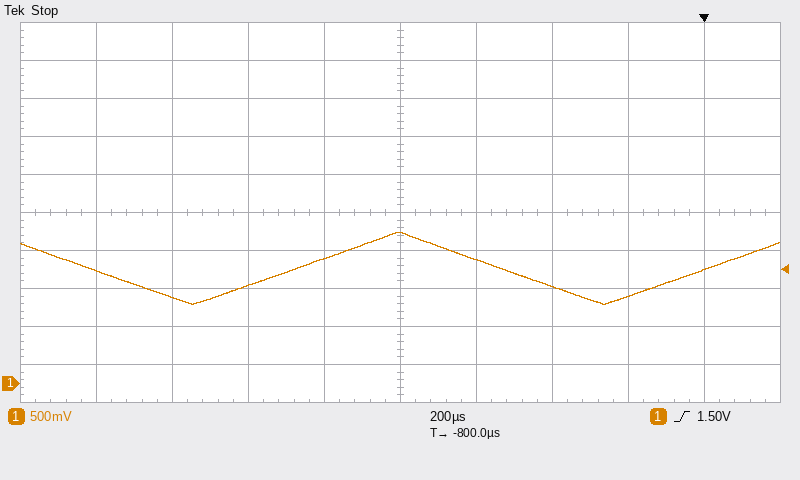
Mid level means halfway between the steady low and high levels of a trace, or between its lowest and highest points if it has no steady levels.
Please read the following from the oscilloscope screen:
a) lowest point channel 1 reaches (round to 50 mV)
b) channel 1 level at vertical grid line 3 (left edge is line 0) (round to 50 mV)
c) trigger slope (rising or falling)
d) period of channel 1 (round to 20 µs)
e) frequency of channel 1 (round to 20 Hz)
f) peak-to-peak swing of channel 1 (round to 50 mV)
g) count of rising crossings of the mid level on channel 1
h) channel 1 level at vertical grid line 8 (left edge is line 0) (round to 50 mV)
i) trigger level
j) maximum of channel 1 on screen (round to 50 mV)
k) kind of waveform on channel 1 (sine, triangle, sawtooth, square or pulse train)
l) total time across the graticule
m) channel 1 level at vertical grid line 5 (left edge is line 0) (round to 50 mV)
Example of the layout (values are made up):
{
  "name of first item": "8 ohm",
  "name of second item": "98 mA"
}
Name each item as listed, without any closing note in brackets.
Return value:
{
  "lowest point channel 1 reaches": "1.05 V",
  "channel 1 level at vertical grid line 3 (left edge is line 0)": "1.30 V",
  "trigger slope": "rising",
  "period of channel 1": "1.08 ms",
  "frequency of channel 1": "920 Hz",
  "peak-to-peak swing of channel 1": "950 mV",
  "count of rising crossings of the mid level on channel 1": "2",
  "channel 1 level at vertical grid line 8 (left edge is line 0)": "1.15 V",
  "trigger level": "1.50 V",
  "maximum of channel 1 on screen": "2.00 V",
  "kind of waveform on channel 1": "triangle",
  "total time across the graticule": "2 ms",
  "channel 1 level at vertical grid line 5 (left edge is line 0)": "2.00 V"
}
